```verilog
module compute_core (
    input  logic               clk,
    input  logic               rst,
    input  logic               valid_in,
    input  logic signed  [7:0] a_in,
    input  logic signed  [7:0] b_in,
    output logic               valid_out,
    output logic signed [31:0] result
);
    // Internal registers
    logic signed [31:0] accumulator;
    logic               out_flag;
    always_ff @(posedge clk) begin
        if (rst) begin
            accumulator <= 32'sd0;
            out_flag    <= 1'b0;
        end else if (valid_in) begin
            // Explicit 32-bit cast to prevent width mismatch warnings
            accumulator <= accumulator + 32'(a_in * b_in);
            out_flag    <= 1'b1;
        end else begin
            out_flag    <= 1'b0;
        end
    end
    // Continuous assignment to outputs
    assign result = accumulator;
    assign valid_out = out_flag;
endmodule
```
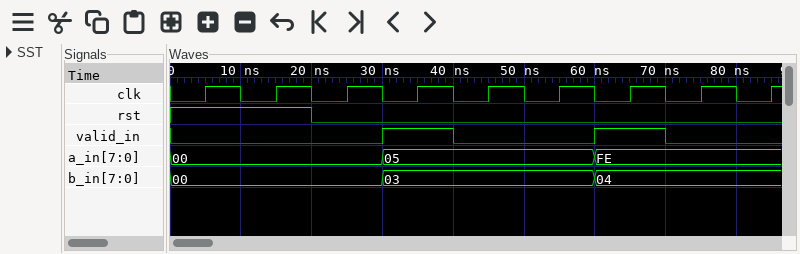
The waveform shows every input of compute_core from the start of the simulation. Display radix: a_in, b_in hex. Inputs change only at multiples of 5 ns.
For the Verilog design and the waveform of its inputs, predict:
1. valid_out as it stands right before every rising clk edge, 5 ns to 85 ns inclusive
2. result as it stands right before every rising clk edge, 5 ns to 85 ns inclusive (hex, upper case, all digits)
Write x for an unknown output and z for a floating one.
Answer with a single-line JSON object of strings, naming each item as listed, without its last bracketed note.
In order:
{"valid_out as it stands right before every rising clk edge, 5 ns to 85 ns inclusive": "x 0 0 0 1 0 0 1 0", "result as it stands right before every rising clk edge, 5 ns to 85 ns inclusive": "x, 00000000, 00000000, 00000000, 0000000F, 0000000F, 0000000F, 00000007, 00000007"}
